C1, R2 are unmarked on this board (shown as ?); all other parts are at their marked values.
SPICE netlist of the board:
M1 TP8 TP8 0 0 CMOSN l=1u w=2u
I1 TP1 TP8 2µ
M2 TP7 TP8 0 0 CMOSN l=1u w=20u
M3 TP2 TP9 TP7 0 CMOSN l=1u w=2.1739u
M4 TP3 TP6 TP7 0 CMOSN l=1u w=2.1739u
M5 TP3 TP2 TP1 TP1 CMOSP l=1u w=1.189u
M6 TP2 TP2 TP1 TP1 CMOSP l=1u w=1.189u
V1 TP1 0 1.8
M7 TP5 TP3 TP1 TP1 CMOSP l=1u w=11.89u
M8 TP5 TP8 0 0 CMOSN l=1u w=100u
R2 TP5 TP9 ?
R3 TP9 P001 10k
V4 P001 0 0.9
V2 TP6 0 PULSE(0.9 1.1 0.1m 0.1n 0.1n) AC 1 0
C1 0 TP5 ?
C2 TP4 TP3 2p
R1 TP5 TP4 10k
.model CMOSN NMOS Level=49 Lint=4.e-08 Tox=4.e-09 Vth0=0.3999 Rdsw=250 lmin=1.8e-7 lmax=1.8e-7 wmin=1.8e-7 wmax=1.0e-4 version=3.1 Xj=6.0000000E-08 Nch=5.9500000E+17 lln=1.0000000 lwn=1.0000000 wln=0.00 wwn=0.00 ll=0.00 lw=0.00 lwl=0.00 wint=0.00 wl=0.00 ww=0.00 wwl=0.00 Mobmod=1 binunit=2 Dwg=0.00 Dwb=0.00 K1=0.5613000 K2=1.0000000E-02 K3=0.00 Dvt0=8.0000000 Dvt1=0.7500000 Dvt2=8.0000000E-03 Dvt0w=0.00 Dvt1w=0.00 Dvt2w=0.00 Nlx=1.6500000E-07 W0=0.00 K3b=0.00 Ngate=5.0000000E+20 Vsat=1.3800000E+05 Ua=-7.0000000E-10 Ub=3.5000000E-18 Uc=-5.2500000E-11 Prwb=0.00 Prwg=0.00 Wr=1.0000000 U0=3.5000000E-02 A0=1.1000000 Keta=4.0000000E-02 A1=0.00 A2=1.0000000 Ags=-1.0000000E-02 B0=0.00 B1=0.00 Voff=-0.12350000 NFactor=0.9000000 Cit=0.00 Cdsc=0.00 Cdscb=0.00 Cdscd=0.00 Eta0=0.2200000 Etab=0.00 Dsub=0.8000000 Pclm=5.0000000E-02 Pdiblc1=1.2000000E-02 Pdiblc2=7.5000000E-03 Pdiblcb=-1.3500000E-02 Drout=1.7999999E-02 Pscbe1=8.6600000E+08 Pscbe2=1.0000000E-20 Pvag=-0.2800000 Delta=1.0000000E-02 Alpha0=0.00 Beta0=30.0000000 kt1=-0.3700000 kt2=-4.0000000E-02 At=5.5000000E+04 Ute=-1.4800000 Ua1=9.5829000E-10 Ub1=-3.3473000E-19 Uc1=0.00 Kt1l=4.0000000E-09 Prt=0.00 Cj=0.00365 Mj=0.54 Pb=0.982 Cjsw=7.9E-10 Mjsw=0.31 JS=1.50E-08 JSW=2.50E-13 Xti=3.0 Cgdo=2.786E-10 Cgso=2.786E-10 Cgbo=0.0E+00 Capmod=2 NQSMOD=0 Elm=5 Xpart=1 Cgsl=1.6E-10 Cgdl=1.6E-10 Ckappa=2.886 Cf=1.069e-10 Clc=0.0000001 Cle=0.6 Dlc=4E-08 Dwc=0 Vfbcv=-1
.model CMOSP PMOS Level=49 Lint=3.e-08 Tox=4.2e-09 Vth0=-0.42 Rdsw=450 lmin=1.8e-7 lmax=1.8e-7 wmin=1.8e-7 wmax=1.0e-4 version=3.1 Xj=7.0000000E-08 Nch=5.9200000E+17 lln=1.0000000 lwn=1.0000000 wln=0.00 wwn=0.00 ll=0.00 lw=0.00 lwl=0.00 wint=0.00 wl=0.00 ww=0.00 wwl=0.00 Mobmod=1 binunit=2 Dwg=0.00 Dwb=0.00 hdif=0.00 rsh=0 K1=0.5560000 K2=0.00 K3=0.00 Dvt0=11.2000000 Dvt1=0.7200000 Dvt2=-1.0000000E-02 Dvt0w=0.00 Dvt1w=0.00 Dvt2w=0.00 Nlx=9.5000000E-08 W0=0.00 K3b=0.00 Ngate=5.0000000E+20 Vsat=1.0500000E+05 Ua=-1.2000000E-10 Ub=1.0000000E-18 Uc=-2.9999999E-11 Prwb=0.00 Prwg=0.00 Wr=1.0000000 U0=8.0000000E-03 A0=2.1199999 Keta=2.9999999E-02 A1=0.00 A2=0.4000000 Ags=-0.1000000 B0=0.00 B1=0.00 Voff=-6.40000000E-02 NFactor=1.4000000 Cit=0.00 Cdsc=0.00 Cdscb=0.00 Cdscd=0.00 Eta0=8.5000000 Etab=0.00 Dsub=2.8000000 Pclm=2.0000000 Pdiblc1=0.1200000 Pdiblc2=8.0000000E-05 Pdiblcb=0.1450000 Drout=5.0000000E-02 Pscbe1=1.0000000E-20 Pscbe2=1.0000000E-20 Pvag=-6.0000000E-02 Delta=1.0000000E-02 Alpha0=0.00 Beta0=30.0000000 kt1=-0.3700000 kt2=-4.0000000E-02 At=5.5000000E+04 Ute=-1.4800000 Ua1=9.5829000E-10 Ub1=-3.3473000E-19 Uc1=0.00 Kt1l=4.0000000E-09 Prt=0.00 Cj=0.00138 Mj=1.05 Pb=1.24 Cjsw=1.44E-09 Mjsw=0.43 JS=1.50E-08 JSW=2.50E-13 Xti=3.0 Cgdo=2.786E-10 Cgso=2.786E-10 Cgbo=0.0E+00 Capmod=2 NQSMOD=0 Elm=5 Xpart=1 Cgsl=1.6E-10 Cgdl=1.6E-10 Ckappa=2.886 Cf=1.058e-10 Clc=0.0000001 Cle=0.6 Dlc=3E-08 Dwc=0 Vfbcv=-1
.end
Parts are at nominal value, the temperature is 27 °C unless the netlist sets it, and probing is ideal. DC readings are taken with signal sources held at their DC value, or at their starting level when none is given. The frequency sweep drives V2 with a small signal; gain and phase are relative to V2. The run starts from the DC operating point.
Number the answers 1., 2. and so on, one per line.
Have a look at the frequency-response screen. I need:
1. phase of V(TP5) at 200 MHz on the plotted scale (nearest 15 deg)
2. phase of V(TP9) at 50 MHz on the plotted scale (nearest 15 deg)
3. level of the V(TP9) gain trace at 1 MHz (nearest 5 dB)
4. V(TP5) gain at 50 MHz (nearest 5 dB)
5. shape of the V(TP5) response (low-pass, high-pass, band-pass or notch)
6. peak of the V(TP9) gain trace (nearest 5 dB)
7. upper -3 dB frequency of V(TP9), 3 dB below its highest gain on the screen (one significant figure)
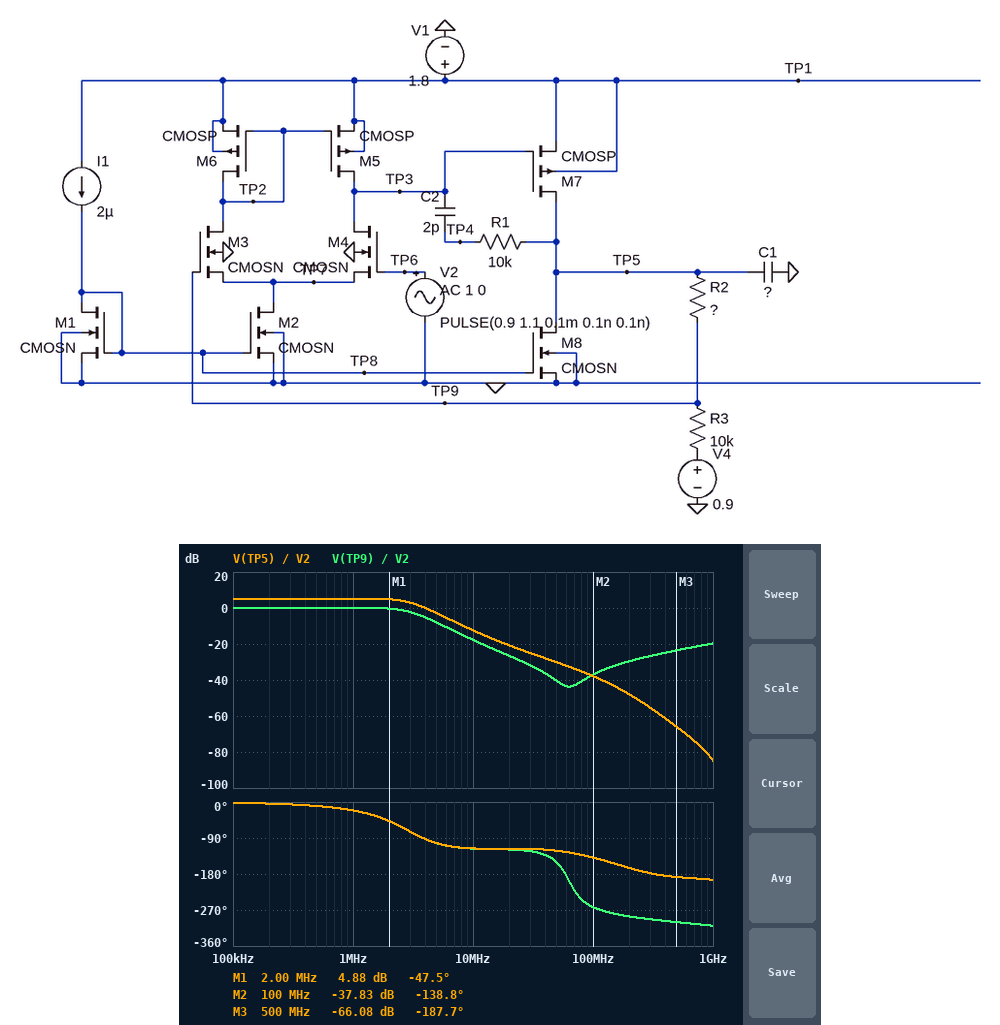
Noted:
1. -165 deg
2. -150 deg
3. 0 dB
4. -30 dB
5. low-pass
6. 0 dB
7. 3 MHz
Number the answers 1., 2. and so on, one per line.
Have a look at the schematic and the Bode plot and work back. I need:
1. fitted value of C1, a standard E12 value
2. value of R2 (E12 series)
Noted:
1. 15 pF
2. 8.2 kΩ
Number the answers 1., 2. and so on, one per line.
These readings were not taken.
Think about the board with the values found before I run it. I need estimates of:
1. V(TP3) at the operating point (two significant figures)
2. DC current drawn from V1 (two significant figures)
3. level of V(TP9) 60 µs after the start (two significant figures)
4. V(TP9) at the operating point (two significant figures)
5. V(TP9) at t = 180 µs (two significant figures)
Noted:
1. 720 mV
2. 130 µA
3. 900 mV
4. 900 mV
5. 1.1 V
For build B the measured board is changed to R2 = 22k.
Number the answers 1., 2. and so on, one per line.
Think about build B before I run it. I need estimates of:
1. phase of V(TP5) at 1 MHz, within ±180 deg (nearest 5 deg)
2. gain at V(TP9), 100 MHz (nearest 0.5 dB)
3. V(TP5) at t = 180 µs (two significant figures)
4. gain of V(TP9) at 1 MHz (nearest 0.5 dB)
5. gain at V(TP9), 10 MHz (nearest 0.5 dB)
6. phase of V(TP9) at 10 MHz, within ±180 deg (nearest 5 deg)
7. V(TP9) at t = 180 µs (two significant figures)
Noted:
1. -35 deg
2. -32.0 dB
3. 1.5 V
4. -0.5 dB
5. -23.0 dB
6. -120 deg
7. 1.1 V
